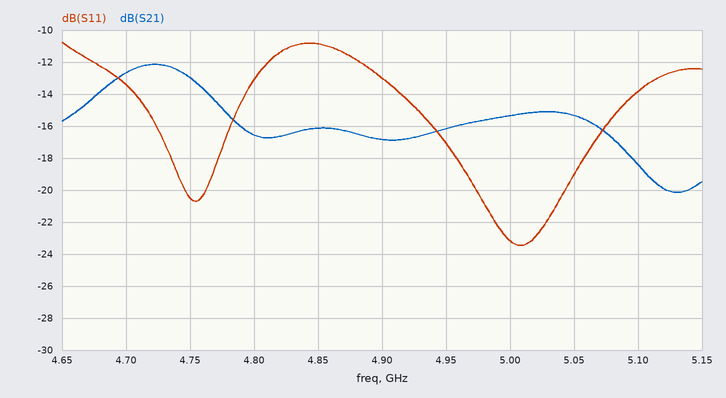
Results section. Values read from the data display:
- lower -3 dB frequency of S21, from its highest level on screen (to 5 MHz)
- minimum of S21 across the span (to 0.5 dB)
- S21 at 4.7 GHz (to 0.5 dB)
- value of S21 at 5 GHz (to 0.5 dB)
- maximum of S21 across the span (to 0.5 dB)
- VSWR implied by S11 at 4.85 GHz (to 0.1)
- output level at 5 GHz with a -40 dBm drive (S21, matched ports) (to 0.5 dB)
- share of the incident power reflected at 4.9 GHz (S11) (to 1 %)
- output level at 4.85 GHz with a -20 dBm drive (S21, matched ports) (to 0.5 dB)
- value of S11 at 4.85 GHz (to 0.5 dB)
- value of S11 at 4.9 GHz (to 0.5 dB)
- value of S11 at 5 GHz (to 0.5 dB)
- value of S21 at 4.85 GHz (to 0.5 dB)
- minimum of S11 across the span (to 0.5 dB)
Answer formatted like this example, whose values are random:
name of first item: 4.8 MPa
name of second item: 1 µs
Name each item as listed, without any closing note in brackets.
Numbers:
lower -3 dB frequency of S21, from its highest level on screen: 4.660 GHz
minimum of S21 across the span: -20.0 dB
S21 at 4.7 GHz: -12.5 dB
value of S21 at 5 GHz: -15.5 dB
maximum of S21 across the span: -12.0 dB
VSWR implied by S11 at 4.85 GHz: 1.8
output level at 5 GHz with a -40 dBm drive (S21, matched ports): -55.5 dBm
share of the incident power reflected at 4.9 GHz (S11): 5 %
output level at 4.85 GHz with a -20 dBm drive (S21, matched ports): -36.0 dBm
value of S11 at 4.85 GHz: -11.0 dB
value of S11 at 4.9 GHz: -13.0 dB
value of S11 at 5 GHz: -23.0 dB
value of S21 at 4.85 GHz: -16.0 dB
minimum of S11 across the span: -23.5 dB
